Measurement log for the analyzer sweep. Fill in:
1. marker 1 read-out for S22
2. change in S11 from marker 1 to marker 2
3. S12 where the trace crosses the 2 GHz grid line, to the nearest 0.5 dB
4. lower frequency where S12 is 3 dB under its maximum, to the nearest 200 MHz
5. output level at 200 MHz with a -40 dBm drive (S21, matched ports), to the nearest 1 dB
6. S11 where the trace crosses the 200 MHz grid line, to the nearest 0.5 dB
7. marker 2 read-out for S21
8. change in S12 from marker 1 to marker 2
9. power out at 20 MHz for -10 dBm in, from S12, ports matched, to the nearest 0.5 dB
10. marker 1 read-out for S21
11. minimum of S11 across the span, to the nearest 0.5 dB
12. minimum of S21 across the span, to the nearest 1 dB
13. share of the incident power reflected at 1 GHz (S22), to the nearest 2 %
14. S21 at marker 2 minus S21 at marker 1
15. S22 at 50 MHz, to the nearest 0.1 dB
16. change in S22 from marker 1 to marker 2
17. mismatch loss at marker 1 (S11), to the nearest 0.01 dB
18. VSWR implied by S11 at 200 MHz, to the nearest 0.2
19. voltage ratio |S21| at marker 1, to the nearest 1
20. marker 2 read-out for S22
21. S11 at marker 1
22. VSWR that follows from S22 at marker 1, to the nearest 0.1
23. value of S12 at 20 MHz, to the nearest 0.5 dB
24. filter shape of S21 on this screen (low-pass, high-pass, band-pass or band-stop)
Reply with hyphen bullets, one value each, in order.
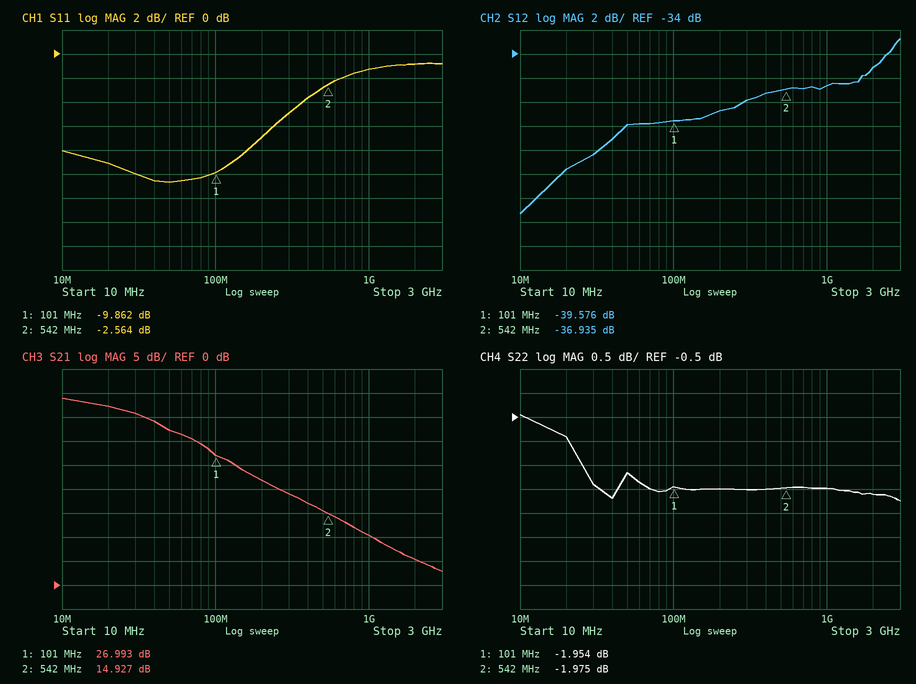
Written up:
- -1.954 dB
- 7.298 dB
- -35.0 dB
- 1.8 GHz
- -18 dBm
- -7.0 dB
- 14.927 dB
- 2.641 dB
- -53.5 dBm
- 26.993 dB
- -10.5 dB
- 3 dB
- 64 %
- -12.066 dB
- -1.7 dB
- -0.021 dB
- 0.47 dB
- 2.6
- 22
- -1.975 dB
- -9.862 dB
- 8.9
- -43.5 dB
- low-pass
